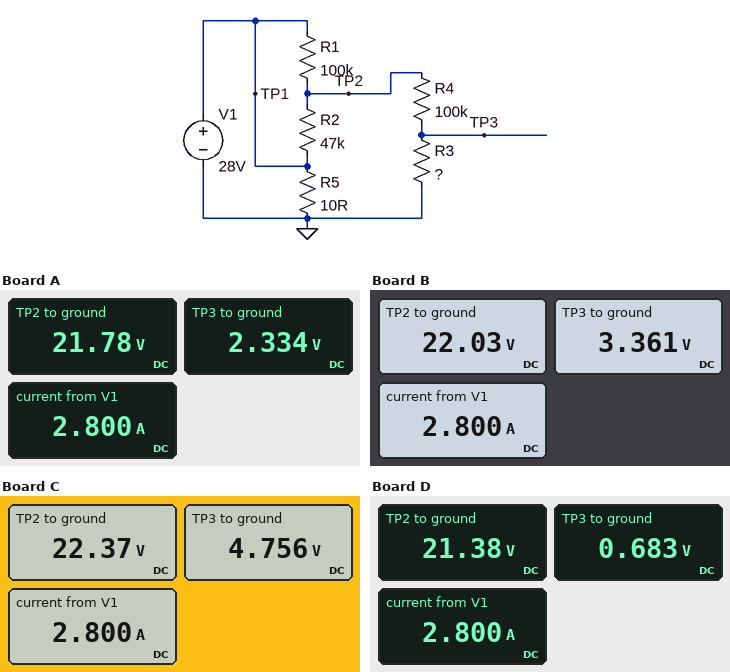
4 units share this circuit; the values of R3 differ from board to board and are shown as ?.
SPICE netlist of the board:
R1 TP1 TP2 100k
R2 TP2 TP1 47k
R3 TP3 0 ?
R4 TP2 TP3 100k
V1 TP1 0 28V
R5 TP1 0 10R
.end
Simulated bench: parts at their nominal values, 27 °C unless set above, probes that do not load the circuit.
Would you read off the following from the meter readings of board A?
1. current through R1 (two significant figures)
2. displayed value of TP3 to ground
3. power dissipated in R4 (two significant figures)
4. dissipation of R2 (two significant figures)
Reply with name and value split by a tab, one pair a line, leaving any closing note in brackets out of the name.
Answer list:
current through R1	62 µA
displayed value of TP3 to ground	2.334 V
power dissipated in R4	3.8 mW
dissipation of R2	820 µW
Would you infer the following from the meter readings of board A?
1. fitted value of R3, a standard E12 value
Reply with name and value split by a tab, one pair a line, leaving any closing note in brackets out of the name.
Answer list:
fitted value of R3, a standard E12 value	12 kΩ
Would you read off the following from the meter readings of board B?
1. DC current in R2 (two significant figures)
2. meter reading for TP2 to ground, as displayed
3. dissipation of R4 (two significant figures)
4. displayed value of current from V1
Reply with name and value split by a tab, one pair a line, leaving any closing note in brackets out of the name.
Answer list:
DC current in R2	130 µA
meter reading for TP2 to ground, as displayed	22.03 V
dissipation of R4	3.5 mW
displayed value of current from V1	2.800 A
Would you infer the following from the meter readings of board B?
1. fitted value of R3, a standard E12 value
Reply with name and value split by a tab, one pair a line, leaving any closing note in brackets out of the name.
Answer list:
fitted value of R3, a standard E12 value	18 kΩ
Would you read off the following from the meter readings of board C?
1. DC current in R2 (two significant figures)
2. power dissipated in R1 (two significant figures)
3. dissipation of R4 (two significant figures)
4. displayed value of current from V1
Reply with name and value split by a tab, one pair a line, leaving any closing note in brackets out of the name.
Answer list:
DC current in R2	120 µA
power dissipated in R1	320 µW
dissipation of R4	3.1 mW
displayed value of current from V1	2.800 A
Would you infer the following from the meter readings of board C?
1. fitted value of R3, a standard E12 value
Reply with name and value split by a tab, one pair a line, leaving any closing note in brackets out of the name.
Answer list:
fitted value of R3, a standard E12 value	27 kΩ
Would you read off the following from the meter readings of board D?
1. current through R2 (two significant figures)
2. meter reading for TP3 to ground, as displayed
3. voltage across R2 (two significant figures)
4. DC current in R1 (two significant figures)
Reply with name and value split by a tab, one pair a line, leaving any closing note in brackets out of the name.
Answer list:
current through R2	140 µA
meter reading for TP3 to ground, as displayed	0.683 V
voltage across R2	6.6 V
DC current in R1	66 µA
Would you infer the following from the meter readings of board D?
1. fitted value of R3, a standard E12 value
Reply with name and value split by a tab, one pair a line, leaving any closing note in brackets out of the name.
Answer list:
fitted value of R3, a standard E12 value	3.3 kΩ
